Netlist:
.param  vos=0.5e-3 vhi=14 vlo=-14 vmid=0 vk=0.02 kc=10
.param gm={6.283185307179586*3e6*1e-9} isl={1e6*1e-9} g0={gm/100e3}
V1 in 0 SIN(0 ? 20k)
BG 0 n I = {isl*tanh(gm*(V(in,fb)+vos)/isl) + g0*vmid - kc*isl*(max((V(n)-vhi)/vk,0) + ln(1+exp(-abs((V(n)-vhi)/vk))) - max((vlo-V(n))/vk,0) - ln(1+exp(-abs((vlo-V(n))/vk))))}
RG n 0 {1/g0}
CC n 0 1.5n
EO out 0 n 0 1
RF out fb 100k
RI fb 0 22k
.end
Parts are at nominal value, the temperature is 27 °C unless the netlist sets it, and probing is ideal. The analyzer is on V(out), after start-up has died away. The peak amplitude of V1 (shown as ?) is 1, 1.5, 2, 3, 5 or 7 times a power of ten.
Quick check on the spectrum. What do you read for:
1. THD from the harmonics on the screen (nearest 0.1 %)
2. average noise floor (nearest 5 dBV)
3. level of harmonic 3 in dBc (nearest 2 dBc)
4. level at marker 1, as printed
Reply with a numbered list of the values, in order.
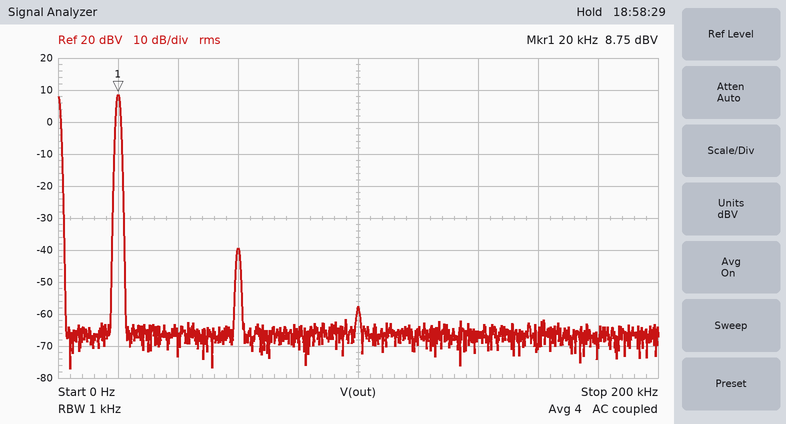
1. 0.4 %
2. -65 dBV
3. -48 dBc
4. 8.75 dBV
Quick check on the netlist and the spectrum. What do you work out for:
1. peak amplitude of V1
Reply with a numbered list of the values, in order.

1. 700 mV
